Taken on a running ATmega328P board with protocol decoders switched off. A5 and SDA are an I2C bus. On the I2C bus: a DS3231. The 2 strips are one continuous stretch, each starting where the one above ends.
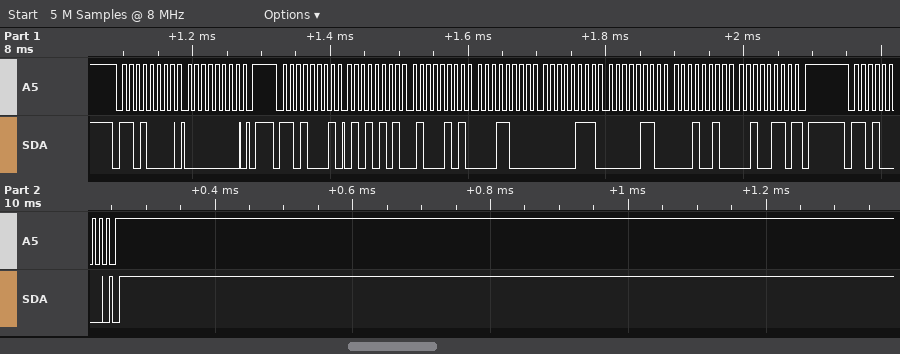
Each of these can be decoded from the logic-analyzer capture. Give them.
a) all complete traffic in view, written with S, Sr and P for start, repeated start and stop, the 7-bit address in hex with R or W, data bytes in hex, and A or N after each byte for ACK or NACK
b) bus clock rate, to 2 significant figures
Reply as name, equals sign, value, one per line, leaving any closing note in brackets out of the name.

all complete traffic in view, written with S, Sr and P for start, repeated start and stop, the 7-bit address in hex with R or W, data bytes in hex, and A or N after each byte for ACK or NACK = S 68W A 00 A P S 68R A 55 A 45 A 18 A 07 A 06 A 12 A 26 N P S 68W A P
bus clock rate, to 2 significant figures = 100 kHz
